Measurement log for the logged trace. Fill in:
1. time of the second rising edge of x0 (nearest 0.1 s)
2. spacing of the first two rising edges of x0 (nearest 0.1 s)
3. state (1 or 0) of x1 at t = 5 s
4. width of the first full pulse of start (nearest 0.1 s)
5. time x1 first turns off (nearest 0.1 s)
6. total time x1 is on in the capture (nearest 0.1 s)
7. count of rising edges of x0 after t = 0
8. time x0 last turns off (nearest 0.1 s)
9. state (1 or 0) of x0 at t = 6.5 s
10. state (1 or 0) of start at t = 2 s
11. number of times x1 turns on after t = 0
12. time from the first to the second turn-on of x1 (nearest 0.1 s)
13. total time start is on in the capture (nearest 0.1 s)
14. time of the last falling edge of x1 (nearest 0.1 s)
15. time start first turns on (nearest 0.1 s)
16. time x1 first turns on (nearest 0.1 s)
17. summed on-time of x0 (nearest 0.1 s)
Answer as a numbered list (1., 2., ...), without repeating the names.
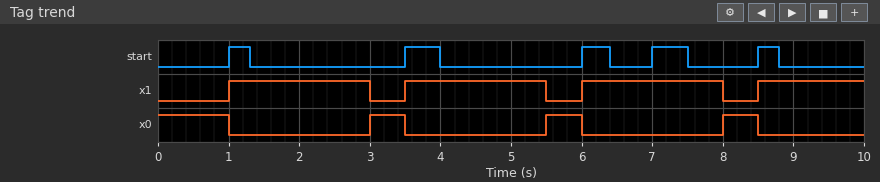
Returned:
1. 5.5 s
2. 2.5 s
3. 1
4. 0.3 s
5. 3.0 s
6. 7.5 s
7. 3
8. 8.5 s
9. 0
10. 0
11. 4
12. 2.5 s
13. 2.0 s
14. 8.0 s
15. 1.0 s
16. 1.0 s
17. 2.5 s
